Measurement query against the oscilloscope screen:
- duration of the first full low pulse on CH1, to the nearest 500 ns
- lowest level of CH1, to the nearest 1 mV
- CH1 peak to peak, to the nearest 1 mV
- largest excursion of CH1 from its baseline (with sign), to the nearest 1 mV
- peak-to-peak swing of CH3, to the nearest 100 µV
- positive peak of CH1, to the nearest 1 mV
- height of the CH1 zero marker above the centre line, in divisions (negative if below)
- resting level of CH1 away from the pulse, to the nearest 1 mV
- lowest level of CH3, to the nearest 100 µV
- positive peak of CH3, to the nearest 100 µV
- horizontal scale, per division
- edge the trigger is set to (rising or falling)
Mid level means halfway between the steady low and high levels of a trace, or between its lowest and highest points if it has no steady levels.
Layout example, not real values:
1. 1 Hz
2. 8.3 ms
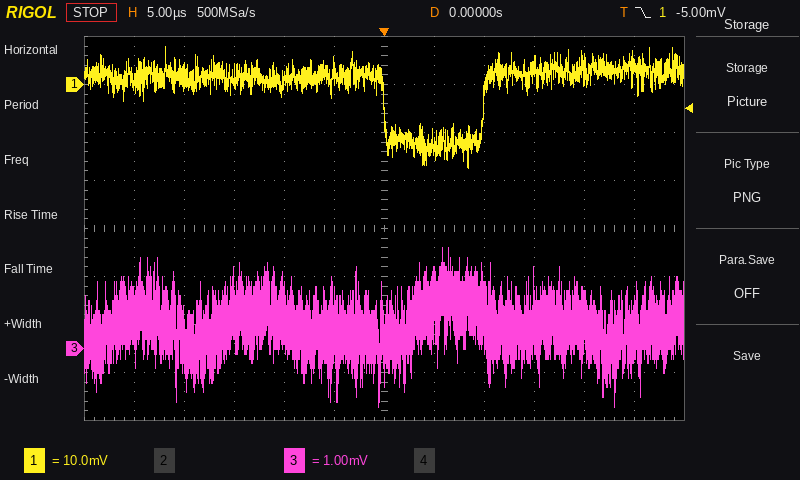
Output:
1. 10.0 µs
2. -17 mV
3. 25 mV
4. -19 mV
5. 3.3 mV
6. 8 mV
7. +3.0 div
8. 2 mV
9. -1.2 mV
10. 2.1 mV
11. 5 µs
12. falling
